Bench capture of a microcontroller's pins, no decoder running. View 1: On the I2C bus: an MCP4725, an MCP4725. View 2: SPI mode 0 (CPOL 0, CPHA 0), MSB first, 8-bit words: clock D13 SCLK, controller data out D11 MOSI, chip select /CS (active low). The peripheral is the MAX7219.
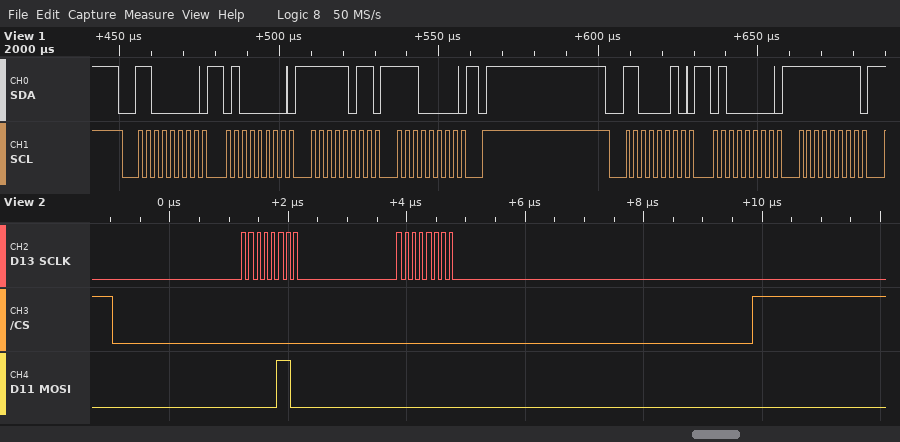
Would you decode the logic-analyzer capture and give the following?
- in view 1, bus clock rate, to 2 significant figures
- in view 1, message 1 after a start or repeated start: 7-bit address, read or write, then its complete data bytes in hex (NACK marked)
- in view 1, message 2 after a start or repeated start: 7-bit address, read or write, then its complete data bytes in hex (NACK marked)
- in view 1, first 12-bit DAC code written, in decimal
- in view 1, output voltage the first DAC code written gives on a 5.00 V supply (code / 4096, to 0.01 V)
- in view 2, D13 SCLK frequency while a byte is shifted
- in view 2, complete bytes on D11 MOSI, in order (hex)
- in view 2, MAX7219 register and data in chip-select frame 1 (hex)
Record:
400 kHz
0x60 write: 40 FB E0
0x61 write: 40 FF
4030
4.92 V
8 MHz
06 00
register 0x6, data 0x00
